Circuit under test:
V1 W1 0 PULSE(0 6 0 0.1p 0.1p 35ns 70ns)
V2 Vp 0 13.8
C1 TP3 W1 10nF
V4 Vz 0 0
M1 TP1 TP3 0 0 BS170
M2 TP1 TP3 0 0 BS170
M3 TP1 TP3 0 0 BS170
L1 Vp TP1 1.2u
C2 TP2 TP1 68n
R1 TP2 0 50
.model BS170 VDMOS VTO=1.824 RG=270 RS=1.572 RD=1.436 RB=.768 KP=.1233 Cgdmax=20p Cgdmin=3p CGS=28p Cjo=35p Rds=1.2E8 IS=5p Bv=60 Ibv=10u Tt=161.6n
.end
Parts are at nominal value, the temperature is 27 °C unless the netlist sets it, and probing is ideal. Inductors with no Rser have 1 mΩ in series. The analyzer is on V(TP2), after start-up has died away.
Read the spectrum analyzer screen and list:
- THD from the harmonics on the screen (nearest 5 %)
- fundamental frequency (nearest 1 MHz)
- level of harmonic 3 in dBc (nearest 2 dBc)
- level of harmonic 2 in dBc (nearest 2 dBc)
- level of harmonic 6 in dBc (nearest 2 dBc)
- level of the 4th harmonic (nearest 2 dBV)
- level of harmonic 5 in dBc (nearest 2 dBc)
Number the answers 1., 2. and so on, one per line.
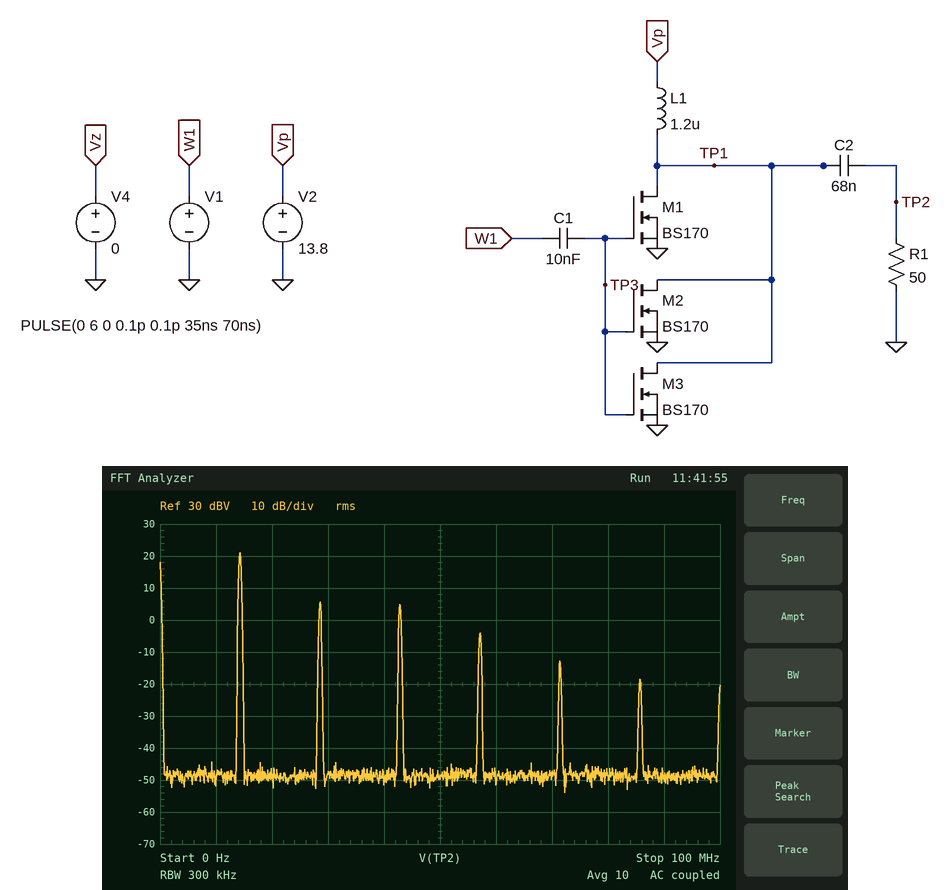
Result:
1. 25 %
2. 14 MHz
3. -16 dBc
4. -16 dBc
5. -40 dBc
6. -4 dBV
7. -34 dBc
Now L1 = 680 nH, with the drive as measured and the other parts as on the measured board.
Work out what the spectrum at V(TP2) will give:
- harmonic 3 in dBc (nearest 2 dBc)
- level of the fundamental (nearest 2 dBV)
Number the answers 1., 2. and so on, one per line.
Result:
1. -14 dBc
2. 22 dBV
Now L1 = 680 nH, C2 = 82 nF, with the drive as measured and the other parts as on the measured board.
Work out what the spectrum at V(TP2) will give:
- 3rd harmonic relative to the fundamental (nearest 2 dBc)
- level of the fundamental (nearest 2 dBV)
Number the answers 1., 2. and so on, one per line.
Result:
1. -14 dBc
2. 22 dBV
